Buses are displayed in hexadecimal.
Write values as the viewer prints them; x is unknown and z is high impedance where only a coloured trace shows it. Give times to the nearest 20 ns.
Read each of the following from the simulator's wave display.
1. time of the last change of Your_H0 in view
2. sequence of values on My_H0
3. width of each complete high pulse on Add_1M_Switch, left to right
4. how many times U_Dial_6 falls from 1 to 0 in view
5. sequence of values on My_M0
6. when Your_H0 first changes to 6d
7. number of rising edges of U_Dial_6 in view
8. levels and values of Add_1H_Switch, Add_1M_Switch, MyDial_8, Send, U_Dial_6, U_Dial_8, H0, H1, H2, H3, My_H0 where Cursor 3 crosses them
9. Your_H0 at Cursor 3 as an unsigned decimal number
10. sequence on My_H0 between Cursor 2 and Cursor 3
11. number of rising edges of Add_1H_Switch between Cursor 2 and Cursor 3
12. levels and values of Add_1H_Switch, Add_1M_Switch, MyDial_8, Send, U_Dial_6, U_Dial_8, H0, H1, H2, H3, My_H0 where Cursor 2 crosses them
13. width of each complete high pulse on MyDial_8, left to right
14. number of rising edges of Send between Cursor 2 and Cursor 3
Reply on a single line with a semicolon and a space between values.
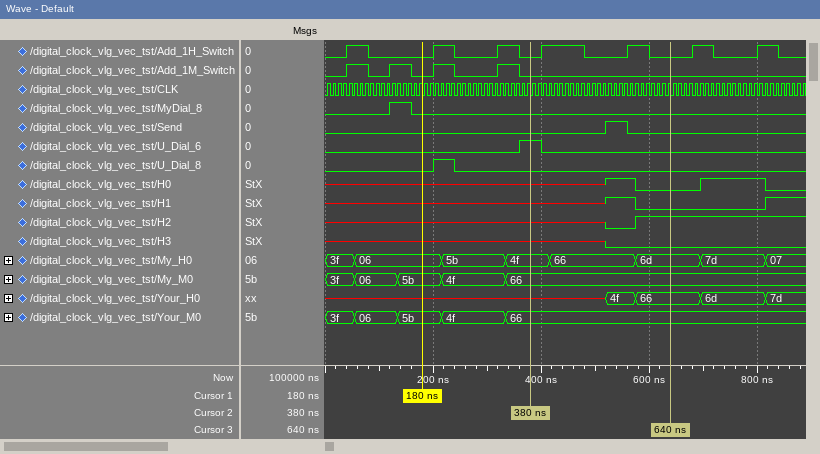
820 ns; 3f, 06, 5b, 4f, 66, 6d, 7d, 07; 40 ns, 40 ns, 40 ns, 40 ns; 1; 3f, 06, 5b, 4f, 66; 700 ns; 1; Add_1H_Switch=0, Add_1M_Switch=0, MyDial_8=0, Send=0, U_Dial_6=0, U_Dial_8=0, H0=0, H1=0, H2=1, H3=0, My_H0=6d; 102; 4f, 66, 6d; 2; Add_1H_Switch=0, Add_1M_Switch=0, MyDial_8=0, Send=0, U_Dial_6=1, U_Dial_8=0, H0=x, H1=x, H2=x, H3=x, My_H0=4f; 40 ns; 1
